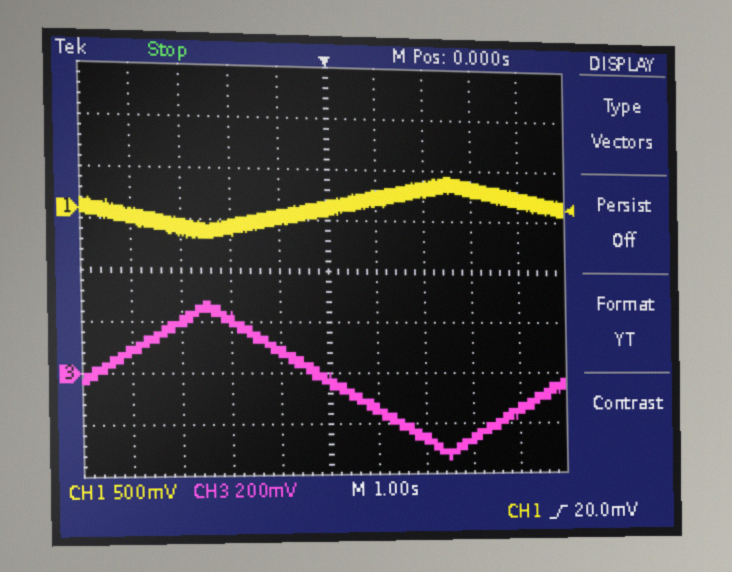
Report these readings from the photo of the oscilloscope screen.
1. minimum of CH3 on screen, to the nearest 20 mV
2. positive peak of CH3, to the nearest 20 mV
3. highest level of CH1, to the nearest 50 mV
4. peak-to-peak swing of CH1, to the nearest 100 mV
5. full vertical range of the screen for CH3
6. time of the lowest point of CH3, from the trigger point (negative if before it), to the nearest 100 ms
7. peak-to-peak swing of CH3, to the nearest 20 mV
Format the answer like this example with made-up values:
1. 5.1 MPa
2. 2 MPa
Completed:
1. -340 mV
2. 280 mV
3. 350 mV
4. 600 mV
5. 1.6 V
6. +2.5 s
7. 620 mV
